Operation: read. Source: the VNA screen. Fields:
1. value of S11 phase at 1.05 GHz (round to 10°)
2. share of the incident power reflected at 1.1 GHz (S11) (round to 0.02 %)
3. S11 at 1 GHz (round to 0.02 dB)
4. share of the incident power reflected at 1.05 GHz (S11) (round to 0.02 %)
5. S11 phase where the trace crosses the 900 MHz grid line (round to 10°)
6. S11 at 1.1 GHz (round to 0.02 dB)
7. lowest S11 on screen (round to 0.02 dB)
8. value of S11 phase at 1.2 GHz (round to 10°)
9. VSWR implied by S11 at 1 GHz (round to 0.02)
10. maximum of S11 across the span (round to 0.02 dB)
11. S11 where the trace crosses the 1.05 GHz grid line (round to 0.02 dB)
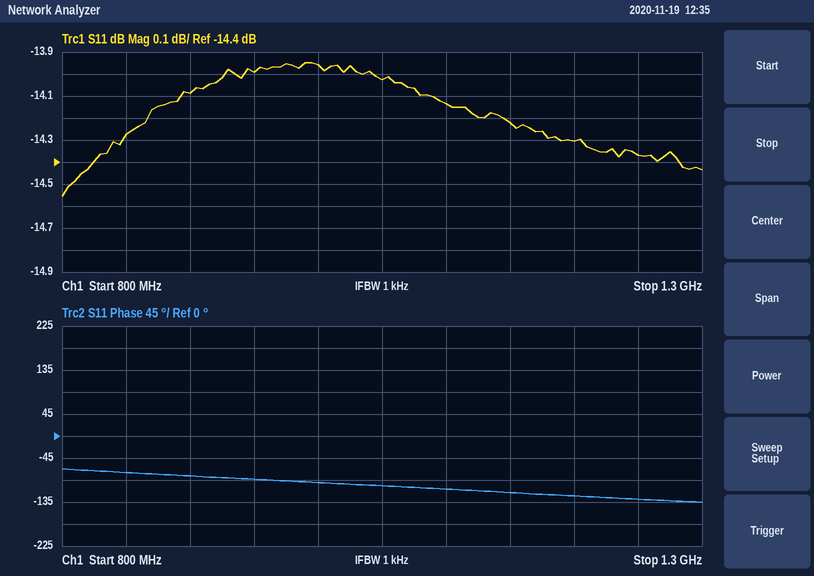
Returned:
-100°
3.86 %
-13.96 dB
3.96 %
-80°
-14.14 dB
-14.56 dB
-120°
1.50
-13.94 dB
-14.02 dB
